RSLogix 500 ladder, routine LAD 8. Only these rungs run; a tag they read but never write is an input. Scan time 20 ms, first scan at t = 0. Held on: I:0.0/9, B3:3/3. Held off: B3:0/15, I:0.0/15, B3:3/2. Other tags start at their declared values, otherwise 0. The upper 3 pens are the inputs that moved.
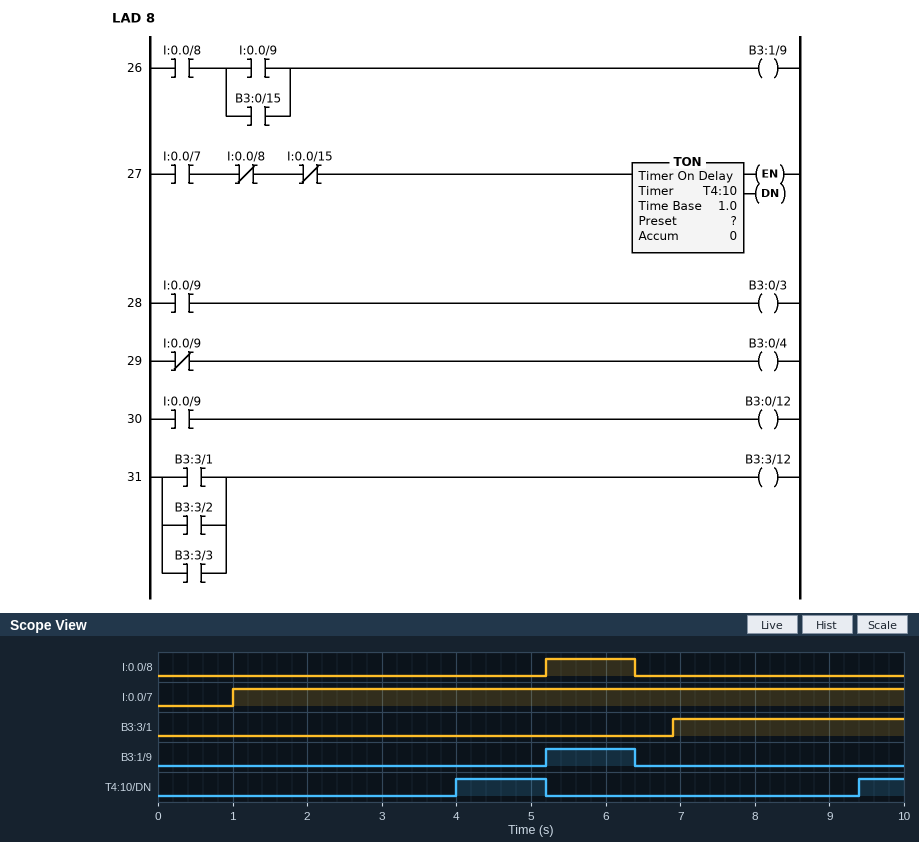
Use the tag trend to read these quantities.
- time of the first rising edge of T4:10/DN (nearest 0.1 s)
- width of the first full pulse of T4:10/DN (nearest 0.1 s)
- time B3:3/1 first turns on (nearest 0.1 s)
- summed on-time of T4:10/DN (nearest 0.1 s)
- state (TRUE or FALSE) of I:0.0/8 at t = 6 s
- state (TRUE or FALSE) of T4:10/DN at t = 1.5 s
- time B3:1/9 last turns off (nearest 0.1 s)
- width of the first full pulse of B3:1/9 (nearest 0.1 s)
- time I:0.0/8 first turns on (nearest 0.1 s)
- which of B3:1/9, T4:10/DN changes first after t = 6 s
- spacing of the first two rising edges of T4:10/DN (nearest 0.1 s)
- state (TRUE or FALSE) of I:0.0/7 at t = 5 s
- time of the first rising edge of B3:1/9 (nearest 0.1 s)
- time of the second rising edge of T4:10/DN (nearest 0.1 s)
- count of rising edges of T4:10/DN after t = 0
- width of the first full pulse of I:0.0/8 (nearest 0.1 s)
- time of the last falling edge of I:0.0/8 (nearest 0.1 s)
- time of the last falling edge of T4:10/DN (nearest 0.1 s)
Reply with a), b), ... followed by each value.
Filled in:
a) 4.0 s
b) 1.2 s
c) 6.9 s
d) 1.8 s
e) TRUE
f) FALSE
g) 6.4 s
h) 1.2 s
i) 5.2 s
j) B3:1/9
k) 5.4 s
l) TRUE
m) 5.2 s
n) 9.4 s
o) 2
p) 1.2 s
q) 6.4 s
r) 5.2 s
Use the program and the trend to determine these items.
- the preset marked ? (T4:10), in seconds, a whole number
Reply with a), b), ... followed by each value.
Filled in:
a) 3 s
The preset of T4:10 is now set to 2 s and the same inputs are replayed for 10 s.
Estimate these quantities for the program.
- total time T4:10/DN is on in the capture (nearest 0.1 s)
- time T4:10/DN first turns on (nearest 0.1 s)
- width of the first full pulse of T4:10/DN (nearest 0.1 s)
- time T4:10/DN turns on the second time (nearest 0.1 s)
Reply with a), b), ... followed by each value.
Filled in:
a) 3.8 s
b) 3.0 s
c) 2.2 s
d) 8.4 s
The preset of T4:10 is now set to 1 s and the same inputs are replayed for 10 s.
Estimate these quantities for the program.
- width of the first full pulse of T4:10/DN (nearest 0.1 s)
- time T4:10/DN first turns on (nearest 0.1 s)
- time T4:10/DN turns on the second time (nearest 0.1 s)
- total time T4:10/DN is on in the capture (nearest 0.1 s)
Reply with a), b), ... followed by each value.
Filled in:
a) 3.2 s
b) 2.0 s
c) 7.4 s
d) 5.8 s
